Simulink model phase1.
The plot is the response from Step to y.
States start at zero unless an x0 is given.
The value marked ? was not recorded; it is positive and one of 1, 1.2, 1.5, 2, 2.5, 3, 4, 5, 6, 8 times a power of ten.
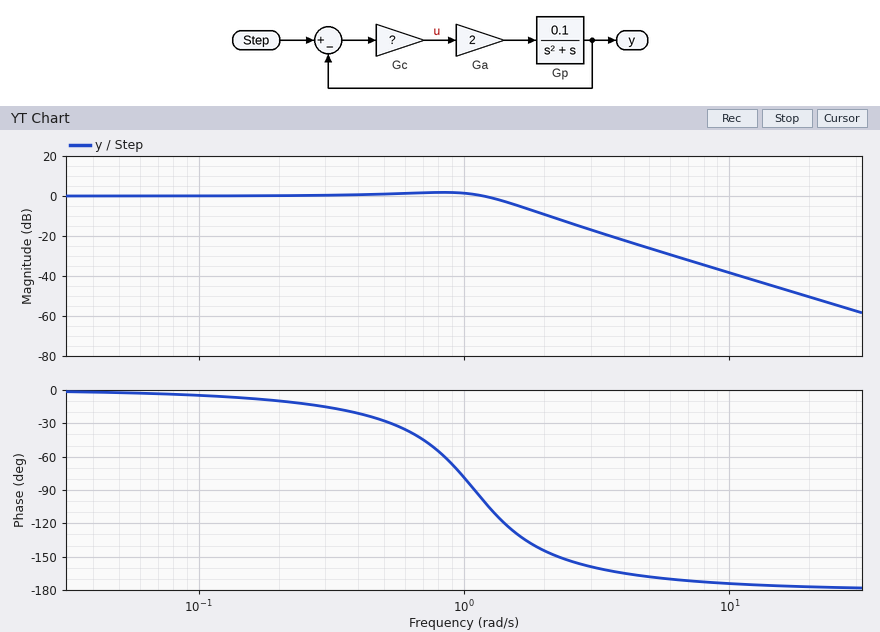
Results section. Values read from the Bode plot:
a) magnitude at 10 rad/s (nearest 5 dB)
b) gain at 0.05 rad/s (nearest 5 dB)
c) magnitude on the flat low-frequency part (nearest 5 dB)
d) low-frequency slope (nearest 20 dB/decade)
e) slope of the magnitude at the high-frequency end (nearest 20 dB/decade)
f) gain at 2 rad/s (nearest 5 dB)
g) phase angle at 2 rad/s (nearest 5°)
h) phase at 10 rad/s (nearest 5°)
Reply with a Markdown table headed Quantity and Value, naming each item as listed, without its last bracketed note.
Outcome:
| Quantity | Value |
|---|---|
| magnitude at 10 rad/s | -40 dB |
| gain at 0.05 rad/s | 0 dB |
| magnitude on the flat low-frequency part | 0 dB |
| low-frequency slope | 0 dB/decade |
| slope of the magnitude at the high-frequency end | -40 dB/decade |
| gain at 2 rad/s | -10 dB |
| phase angle at 2 rad/s | -145° |
| phase at 10 rad/s | -175° |
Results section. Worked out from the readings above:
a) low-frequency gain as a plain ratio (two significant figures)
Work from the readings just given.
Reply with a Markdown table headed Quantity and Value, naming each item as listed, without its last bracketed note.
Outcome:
| Quantity | Value |
|---|---|
| low-frequency gain as a plain ratio | 1.0 |
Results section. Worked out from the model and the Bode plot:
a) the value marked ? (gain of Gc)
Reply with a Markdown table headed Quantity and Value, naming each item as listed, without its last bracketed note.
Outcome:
| Quantity | Value |
|---|---|
| the value marked ? | 6 |
